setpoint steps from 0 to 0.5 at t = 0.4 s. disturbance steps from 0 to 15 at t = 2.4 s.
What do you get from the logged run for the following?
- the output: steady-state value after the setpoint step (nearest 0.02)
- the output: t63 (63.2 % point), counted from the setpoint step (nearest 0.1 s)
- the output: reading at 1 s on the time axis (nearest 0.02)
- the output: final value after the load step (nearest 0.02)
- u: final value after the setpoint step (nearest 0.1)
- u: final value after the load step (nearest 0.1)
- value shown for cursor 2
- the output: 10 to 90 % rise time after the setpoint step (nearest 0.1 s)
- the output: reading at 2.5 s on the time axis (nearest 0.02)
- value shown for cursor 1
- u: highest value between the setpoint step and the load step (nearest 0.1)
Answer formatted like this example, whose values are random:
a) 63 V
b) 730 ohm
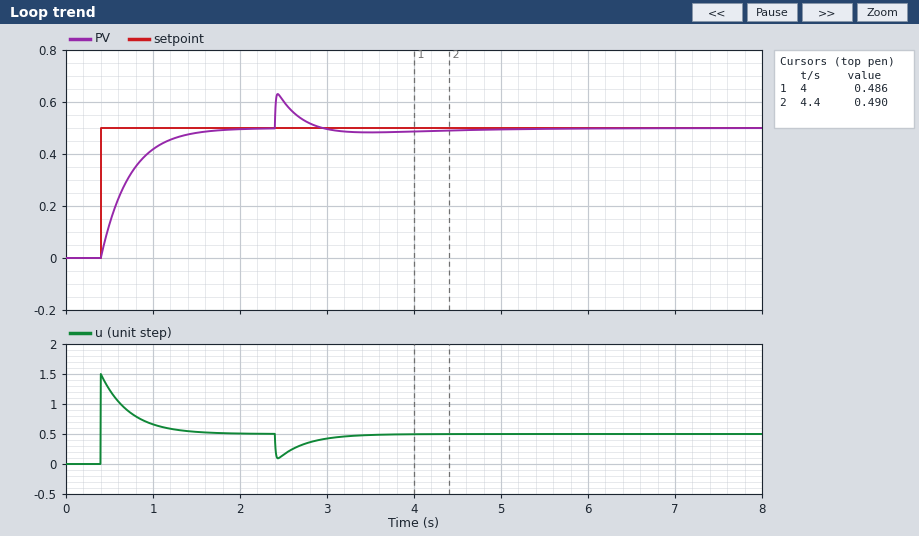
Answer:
a) 0.50
b) 0.3 s
c) 0.42
d) 0.50
e) 0.5
f) 0.5
g) 0.490
h) 0.7 s
i) 0.60
j) 0.486
k) 1.5
